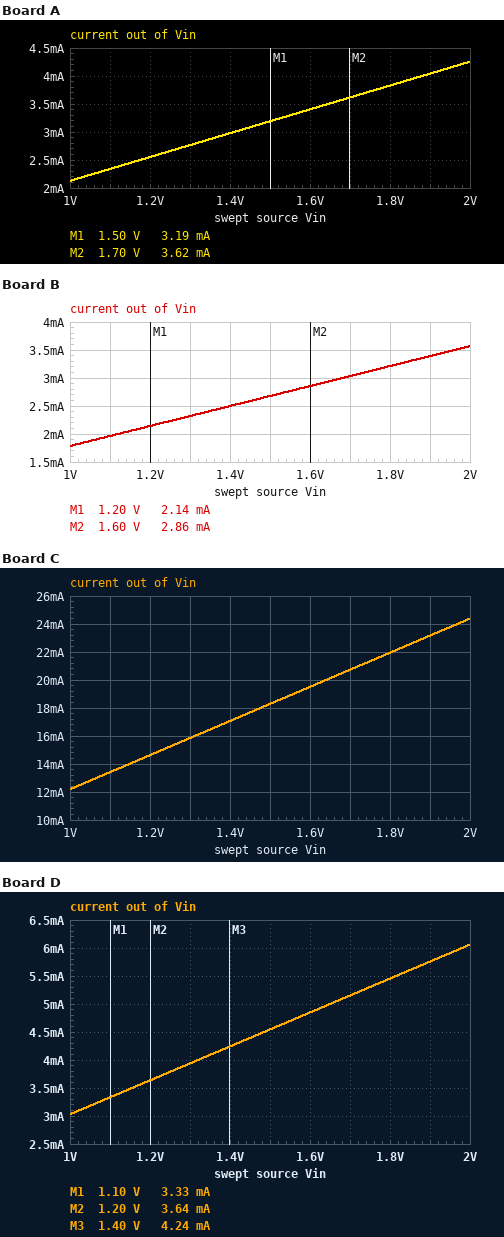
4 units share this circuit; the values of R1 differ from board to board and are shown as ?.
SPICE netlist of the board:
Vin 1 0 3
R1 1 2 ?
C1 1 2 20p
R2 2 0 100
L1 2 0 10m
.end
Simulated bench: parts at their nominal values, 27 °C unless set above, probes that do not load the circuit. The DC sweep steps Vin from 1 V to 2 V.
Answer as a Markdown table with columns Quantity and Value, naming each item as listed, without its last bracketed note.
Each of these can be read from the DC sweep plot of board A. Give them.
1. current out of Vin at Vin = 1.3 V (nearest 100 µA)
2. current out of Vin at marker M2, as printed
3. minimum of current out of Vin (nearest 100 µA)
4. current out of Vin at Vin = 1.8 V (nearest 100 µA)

| Quantity | Value |
|---|---|
| current out of Vin at Vin = 1.3 V | 2.8 mA |
| current out of Vin at marker M2, as printed | 3.62 mA |
| minimum of current out of Vin | 2.1 mA |
| current out of Vin at Vin = 1.8 V | 3.8 mA |
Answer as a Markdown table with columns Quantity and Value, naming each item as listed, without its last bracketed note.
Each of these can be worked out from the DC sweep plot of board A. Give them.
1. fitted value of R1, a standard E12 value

| Quantity | Value |
|---|---|
| fitted value of R1, a standard E12 value | 470 Ω |
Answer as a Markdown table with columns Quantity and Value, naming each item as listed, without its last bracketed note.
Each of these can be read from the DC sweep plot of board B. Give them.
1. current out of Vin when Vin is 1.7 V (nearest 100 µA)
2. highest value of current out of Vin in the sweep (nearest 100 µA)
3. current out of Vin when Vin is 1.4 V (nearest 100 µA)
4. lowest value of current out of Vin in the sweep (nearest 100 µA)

| Quantity | Value |
|---|---|
| current out of Vin when Vin is 1.7 V | 3.0 mA |
| highest value of current out of Vin in the sweep | 3.6 mA |
| current out of Vin when Vin is 1.4 V | 2.5 mA |
| lowest value of current out of Vin in the sweep | 1.8 mA |
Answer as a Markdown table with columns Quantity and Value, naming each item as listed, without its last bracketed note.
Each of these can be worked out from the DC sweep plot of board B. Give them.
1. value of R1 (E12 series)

| Quantity | Value |
|---|---|
| value of R1 | 560 Ω |
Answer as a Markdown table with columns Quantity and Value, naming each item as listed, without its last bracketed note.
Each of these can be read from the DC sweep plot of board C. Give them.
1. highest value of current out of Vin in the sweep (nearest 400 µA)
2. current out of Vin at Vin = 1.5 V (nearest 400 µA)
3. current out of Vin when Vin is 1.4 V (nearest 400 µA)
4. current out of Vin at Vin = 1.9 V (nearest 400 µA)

| Quantity | Value |
|---|---|
| highest value of current out of Vin in the sweep | 24.4 mA |
| current out of Vin at Vin = 1.5 V | 18.4 mA |
| current out of Vin when Vin is 1.4 V | 17.2 mA |
| current out of Vin at Vin = 1.9 V | 23.2 mA |
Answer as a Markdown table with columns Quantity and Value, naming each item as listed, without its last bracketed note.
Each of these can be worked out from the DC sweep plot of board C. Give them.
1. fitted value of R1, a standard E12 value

| Quantity | Value |
|---|---|
| fitted value of R1, a standard E12 value | 82 Ω |
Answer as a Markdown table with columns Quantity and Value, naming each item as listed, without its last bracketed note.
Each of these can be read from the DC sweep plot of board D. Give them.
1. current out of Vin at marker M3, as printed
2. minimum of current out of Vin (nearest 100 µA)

| Quantity | Value |
|---|---|
| current out of Vin at marker M3, as printed | 4.24 mA |
| minimum of current out of Vin | 3.0 mA |
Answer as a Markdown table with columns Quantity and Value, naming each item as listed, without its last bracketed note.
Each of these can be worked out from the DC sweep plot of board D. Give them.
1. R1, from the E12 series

| Quantity | Value |
|---|---|
| R1, from the E12 series | 330 Ω |
